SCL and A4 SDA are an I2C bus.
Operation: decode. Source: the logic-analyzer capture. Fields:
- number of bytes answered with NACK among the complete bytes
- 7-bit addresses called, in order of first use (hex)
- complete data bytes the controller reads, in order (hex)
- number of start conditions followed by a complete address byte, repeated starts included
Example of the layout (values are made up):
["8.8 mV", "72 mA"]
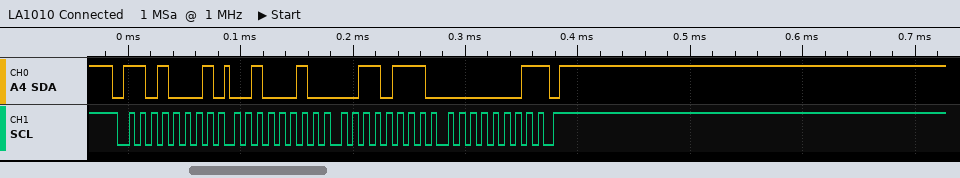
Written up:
["1", "0x68", "22 37 01", "1"]
